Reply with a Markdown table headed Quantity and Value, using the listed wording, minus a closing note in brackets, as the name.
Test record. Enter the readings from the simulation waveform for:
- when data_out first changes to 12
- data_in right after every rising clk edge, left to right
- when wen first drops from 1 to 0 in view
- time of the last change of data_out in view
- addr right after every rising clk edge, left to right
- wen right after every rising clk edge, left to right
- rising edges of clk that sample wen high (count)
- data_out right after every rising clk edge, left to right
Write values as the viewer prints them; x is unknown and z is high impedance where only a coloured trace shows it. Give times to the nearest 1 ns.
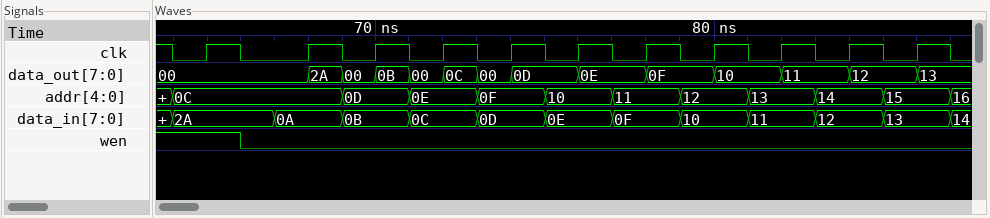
| Quantity | Value |
|---|---|
| when data_out first changes to 12 | 84 ns |
| data_in right after every rising clk edge, left to right | 2A, 0A, 0B, 0C, 0D, 0E, 0F, 10, 11, 12, 13 |
| when wen first drops from 1 to 0 in view | 66 ns |
| time of the last change of data_out in view | 86 ns |
| addr right after every rising clk edge, left to right | 0C, 0C, 0D, 0E, 0F, 10, 11, 12, 13, 14, 15 |
| wen right after every rising clk edge, left to right | 1 0 0 0 0 0 0 0 0 0 0 |
| rising edges of clk that sample wen high | 1 |
| data_out right after every rising clk edge, left to right | 00, 2A, 0B, 0C, 0D, 0E, 0F, 10, 11, 12, 13 |
